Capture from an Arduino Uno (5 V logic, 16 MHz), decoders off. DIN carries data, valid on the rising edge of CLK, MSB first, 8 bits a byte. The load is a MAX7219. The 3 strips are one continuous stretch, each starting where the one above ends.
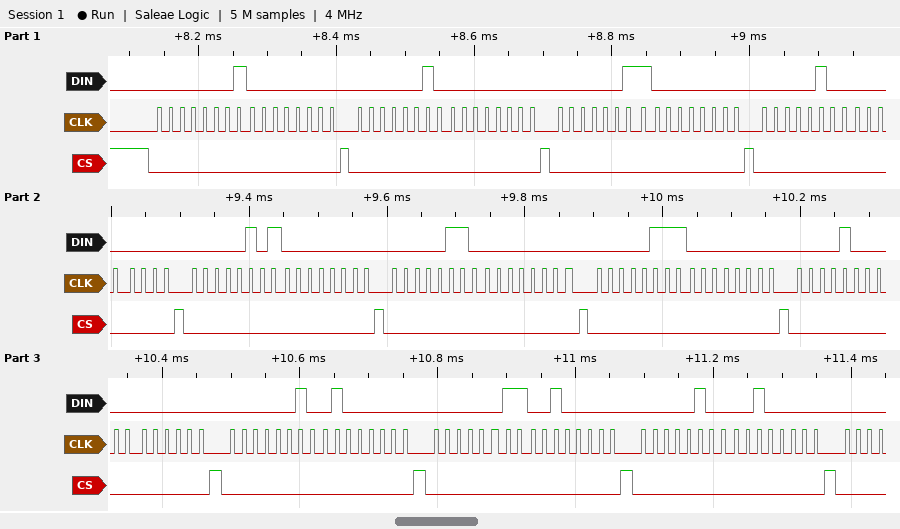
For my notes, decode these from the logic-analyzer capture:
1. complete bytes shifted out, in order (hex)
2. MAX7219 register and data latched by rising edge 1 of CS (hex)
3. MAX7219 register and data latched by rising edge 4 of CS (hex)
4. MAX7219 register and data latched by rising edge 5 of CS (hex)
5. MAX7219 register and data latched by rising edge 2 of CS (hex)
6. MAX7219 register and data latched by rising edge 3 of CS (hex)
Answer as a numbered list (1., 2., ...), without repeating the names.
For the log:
1. 0x01 0x00 0x02 0x00 0x03 0x00 0x04 0x00 0x05 0x00 0x06 0x00 0x07 0x00 0x08 0x00 0x02 0x40 0x03 0x20 0x04 0x20
2. register 0x1, data 0x00
3. register 0x4, data 0x00
4. register 0x5, data 0x00
5. register 0x2, data 0x00
6. register 0x3, data 0x00
